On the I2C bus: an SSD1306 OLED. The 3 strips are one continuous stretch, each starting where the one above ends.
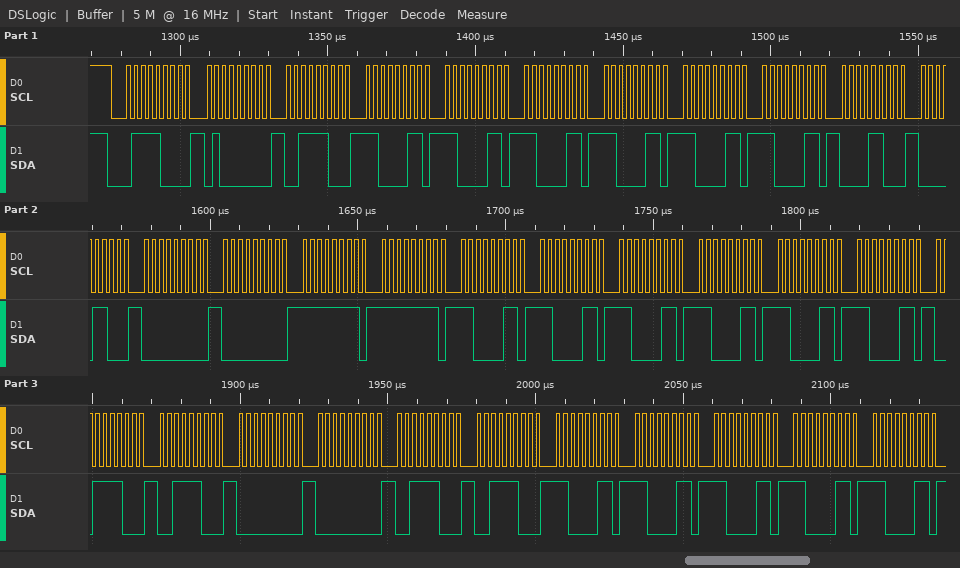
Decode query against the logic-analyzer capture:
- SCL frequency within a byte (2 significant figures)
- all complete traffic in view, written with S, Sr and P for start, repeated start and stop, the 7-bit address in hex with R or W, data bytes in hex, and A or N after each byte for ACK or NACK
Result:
400 kHz
S 3CW A 40 A 3C A C3 A C3 A C3 A C3 A C3 A C3 A 0C A 0C A 00 A 00 A FF A FF A C3 A C3 A C3 A C3 A C3 A C3 A 3C A 3C A 00 A 00 A 3C A 3C A C3 A C3 A C3 A C3 A C3 A
